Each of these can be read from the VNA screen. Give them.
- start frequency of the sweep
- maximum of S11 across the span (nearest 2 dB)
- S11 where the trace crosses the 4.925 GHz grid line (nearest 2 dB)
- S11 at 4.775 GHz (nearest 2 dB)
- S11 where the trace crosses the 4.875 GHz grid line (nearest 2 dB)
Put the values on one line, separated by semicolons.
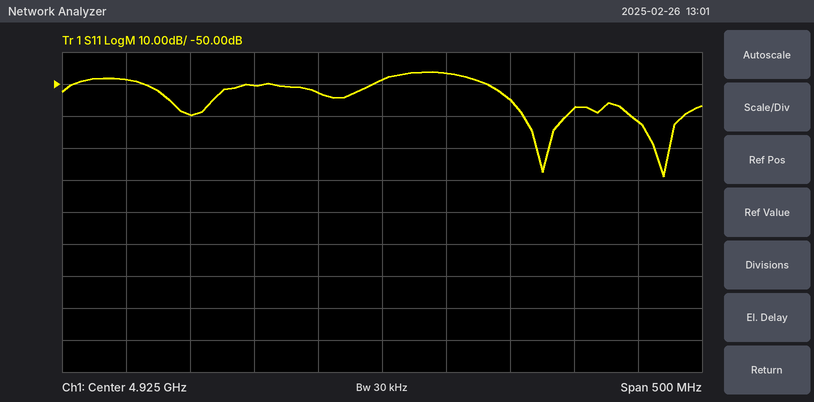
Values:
4.675 GHz; -46 dB; -48 dB; -60 dB; -52 dB
